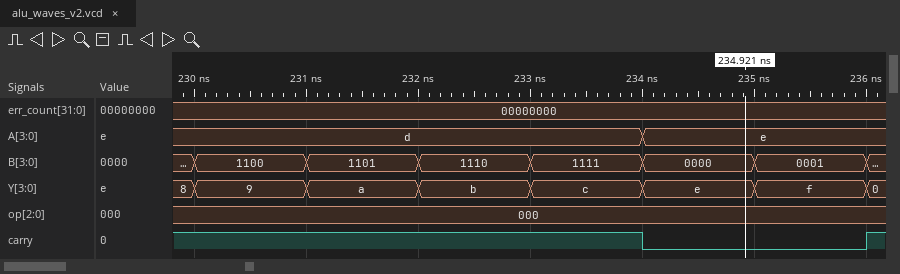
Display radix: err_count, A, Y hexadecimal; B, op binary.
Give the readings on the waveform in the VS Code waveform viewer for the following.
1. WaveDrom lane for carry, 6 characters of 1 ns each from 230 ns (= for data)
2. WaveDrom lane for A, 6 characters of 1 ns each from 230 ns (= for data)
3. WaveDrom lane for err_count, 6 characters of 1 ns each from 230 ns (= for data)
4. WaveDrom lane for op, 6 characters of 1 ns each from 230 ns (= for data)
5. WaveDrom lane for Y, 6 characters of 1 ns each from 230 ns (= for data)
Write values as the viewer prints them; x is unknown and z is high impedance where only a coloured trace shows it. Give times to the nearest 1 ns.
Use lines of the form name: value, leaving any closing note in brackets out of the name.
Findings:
WaveDrom lane for carry, 6 characters of 1 ns each from 230 ns: {name: 'carry', wave: '1...0.'}
WaveDrom lane for A, 6 characters of 1 ns each from 230 ns: {name: 'A', wave: '=...=.', data: 'd e'}
WaveDrom lane for err_count, 6 characters of 1 ns each from 230 ns: {name: 'err_count', wave: '=.....', data: '00000000'}
WaveDrom lane for op, 6 characters of 1 ns each from 230 ns: {name: 'op', wave: '=.....', data: '000'}
WaveDrom lane for Y, 6 characters of 1 ns each from 230 ns: {name: 'Y', wave: '======', data: '9 a b c e f'}
